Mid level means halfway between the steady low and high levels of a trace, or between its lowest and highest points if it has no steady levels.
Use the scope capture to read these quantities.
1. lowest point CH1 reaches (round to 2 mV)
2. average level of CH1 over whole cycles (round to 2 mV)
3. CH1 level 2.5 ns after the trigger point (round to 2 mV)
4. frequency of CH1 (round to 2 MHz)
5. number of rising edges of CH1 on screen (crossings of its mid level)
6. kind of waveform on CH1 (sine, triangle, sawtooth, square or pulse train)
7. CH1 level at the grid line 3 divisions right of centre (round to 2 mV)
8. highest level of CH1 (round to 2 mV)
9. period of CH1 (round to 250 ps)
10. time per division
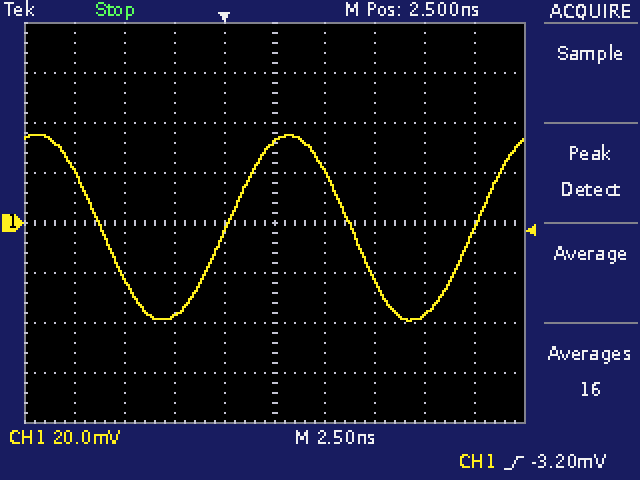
-40 mV
-2 mV
32 mV
80 MHz
2
sine
-36 mV
36 mV
12.50 ns
2.5 ns
